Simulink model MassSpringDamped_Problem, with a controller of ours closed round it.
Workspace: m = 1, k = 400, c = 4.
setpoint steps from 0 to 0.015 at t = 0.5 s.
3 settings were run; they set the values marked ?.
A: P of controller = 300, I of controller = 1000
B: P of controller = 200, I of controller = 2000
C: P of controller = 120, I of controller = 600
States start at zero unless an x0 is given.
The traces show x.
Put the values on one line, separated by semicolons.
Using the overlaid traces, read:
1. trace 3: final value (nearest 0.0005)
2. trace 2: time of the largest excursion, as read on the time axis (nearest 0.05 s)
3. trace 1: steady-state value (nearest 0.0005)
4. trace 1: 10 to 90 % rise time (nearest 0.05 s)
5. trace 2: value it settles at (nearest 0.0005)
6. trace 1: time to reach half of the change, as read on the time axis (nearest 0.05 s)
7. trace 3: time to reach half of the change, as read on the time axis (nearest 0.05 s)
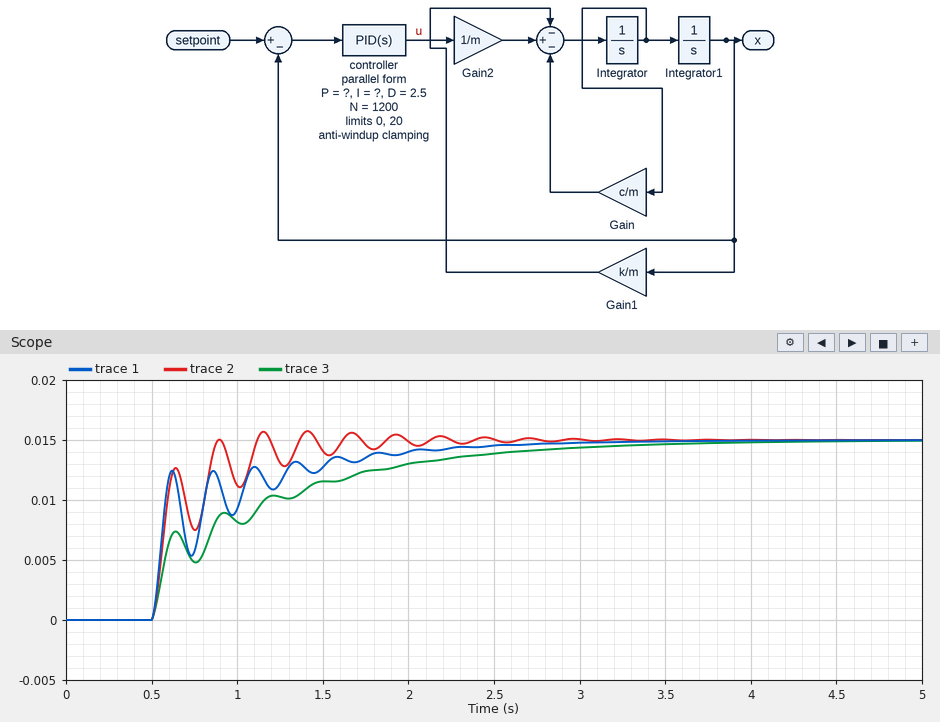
0.0150; 1.40 s; 0.0150; 1.05 s; 0.0150; 0.55 s; 0.85 s
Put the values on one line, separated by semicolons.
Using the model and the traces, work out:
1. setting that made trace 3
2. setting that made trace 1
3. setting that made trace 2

C; A; B
